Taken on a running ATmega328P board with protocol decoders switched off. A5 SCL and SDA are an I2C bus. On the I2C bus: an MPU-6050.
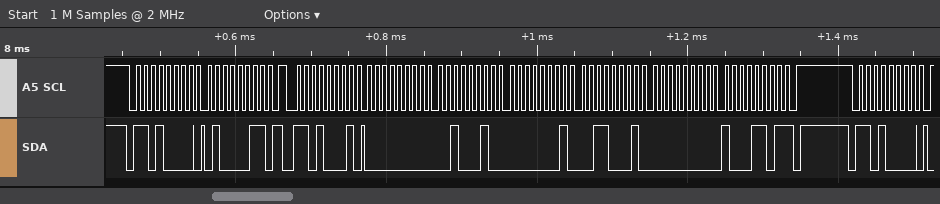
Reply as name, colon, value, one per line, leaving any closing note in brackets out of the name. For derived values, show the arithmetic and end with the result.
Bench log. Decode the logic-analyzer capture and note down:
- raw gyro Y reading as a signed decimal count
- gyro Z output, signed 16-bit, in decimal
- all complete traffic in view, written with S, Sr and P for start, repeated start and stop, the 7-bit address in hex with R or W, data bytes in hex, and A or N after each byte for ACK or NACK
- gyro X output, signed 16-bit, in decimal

raw gyro Y reading as a signed decimal count: 0x0131 = 305
gyro Z output, signed 16-bit, in decimal: 0x008D = 141
all complete traffic in view, written with S, Sr and P for start, repeated start and stop, the 7-bit address in hex with R or W, data bytes in hex, and A or N after each byte for ACK or NACK: S 68W A 43 A Sr 68R A 00 A 22 A 01 A 31 A 00 A 8D N P S 68W A
gyro X output, signed 16-bit, in decimal: 0x0022 = 34
